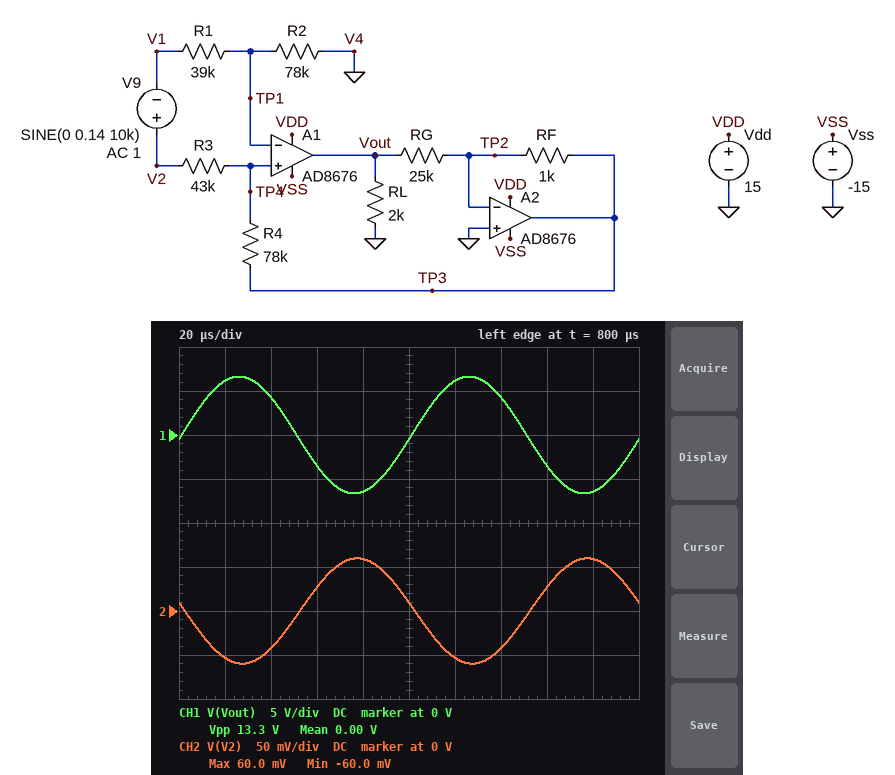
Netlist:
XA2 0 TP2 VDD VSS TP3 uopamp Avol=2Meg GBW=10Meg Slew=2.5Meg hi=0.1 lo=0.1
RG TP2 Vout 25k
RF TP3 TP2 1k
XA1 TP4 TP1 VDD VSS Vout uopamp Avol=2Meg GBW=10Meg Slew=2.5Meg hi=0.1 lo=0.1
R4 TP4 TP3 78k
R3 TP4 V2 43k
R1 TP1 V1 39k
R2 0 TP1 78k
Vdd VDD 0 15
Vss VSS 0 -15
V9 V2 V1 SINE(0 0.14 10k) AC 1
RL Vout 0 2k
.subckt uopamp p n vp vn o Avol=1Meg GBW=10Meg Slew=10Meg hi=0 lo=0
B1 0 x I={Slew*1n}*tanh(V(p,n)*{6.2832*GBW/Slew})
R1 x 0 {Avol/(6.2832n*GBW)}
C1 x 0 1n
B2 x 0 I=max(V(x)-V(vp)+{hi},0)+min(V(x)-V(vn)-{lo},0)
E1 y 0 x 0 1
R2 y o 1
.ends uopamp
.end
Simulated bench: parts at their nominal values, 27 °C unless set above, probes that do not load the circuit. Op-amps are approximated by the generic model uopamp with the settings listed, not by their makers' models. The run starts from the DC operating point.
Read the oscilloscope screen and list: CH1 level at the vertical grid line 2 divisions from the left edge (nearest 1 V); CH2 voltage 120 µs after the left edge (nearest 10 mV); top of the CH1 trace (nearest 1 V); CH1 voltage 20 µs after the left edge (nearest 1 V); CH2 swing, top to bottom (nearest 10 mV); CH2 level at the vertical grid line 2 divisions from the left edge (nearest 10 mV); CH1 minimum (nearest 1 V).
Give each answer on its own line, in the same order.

4 V
-50 mV
7 V
6 V
120 mV
-40 mV
-7 V
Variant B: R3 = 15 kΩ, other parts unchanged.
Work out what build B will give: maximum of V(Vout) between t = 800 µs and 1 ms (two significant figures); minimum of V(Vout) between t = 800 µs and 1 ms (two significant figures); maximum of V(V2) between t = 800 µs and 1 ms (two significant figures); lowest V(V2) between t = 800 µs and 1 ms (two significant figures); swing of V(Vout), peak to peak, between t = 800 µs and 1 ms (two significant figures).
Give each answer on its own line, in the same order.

10 V
-10 V
160 mV
-160 mV
20 V
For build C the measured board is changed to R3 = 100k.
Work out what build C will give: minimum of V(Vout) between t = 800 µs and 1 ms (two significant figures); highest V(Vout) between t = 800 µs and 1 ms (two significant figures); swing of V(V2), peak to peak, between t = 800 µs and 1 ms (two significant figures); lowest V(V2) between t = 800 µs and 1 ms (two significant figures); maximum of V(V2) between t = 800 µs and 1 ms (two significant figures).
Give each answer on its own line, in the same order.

-3.9 V
3.9 V
45 mV
-23 mV
23 mV
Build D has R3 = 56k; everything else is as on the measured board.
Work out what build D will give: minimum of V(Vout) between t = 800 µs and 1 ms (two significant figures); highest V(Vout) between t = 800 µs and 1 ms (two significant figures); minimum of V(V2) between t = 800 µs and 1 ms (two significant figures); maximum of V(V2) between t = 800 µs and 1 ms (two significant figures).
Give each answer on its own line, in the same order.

-5.7 V
5.7 V
-33 mV
33 mV
